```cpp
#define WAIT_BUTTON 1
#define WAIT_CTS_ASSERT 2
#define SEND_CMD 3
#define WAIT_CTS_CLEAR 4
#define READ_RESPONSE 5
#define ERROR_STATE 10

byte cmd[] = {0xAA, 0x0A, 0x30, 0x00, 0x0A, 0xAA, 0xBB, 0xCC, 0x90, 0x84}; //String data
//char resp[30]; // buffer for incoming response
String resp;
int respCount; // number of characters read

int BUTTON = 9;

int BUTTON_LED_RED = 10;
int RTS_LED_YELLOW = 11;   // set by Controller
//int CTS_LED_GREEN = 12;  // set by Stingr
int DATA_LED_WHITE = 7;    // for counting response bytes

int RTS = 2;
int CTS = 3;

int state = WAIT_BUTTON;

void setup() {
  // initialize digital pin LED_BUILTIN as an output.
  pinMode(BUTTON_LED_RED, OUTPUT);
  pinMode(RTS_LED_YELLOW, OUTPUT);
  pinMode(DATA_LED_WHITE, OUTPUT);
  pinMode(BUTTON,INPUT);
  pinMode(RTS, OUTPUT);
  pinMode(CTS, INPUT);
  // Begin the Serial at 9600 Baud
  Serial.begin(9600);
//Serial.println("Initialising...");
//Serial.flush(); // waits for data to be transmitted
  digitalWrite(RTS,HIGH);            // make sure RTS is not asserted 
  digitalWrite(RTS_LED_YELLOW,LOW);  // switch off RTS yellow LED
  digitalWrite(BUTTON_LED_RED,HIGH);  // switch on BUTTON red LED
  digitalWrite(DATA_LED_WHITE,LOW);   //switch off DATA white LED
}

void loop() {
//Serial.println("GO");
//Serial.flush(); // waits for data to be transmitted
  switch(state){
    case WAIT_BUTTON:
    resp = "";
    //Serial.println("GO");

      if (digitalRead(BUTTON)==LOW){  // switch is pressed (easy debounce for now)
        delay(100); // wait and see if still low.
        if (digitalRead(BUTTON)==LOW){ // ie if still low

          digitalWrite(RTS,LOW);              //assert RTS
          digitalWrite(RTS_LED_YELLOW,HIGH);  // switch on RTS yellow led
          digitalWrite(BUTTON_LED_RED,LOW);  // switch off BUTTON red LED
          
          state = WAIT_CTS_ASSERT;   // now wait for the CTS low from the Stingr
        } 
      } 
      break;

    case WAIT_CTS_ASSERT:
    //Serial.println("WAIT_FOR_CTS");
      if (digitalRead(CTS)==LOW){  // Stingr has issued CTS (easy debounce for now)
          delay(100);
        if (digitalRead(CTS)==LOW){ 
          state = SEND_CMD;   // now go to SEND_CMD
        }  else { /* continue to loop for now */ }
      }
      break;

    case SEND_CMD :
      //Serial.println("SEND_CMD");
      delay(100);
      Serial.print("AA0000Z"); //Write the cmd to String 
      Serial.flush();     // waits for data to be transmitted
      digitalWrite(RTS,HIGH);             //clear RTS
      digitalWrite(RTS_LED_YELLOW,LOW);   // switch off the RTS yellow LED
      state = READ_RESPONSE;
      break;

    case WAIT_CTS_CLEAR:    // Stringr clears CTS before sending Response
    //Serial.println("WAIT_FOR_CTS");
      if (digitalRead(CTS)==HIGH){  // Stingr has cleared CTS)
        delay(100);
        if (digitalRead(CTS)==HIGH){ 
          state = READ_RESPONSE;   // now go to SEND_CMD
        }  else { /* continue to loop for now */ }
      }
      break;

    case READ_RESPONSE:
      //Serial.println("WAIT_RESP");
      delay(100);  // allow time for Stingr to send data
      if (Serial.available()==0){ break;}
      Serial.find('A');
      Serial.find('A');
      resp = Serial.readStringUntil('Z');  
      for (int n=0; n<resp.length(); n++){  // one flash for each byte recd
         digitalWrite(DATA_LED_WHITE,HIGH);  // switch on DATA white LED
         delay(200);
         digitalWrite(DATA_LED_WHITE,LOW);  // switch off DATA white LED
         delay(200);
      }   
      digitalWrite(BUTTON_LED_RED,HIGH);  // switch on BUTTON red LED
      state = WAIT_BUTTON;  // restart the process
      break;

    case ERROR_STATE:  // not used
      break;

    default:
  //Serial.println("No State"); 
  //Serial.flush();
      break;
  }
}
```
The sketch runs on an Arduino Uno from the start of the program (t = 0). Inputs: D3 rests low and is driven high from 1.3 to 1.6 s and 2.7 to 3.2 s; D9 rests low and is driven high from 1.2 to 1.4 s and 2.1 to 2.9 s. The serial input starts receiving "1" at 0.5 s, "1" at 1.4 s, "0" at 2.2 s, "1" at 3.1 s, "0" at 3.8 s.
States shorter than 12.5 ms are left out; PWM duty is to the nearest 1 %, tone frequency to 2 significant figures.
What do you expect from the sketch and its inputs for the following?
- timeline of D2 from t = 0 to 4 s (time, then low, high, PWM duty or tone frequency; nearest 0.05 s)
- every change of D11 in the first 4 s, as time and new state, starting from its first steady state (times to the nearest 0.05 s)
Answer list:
0 s high; 0.1 s low; 0.3 s high
0 s low; 0.1 s high; 0.3 s low
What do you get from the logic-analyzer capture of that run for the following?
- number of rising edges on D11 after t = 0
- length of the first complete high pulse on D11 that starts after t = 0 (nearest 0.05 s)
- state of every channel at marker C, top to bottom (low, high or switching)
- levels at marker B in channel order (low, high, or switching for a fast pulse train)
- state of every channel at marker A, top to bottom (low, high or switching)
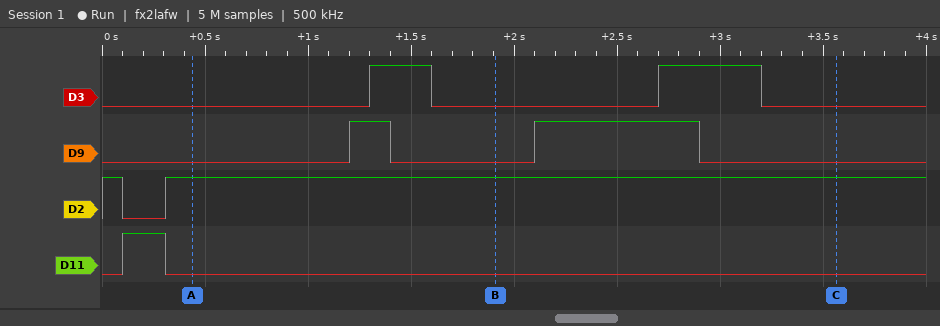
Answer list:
1
0.20 s
D3 low, D9 low, D2 high, D11 low
D3 low, D9 low, D2 high, D11 low
D3 low, D9 low, D2 high, D11 low
